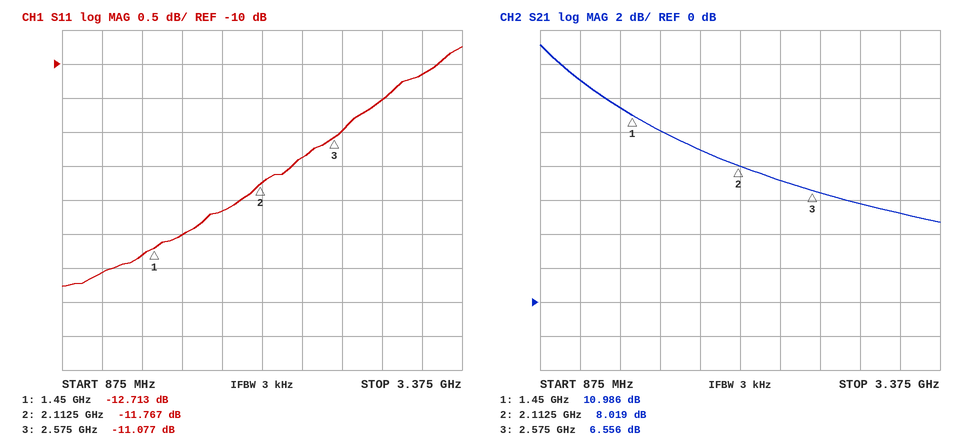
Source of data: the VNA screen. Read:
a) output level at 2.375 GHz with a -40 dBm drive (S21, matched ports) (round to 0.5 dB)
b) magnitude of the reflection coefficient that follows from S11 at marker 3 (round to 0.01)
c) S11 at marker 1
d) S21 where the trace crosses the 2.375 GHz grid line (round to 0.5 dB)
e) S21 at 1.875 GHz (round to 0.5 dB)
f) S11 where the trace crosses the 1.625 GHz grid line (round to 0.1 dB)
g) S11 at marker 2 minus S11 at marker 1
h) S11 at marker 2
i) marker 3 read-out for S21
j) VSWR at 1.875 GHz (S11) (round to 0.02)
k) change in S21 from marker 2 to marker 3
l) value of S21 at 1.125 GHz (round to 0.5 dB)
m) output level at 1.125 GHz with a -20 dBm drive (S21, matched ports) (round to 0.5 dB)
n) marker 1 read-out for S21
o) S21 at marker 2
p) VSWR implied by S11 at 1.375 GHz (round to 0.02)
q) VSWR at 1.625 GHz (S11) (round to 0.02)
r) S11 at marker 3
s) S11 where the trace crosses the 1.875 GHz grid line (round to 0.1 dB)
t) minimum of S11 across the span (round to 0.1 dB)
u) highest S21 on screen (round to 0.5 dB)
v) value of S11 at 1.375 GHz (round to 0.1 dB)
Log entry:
-33.0 dBm
0.28
-12.713 dB
7.0 dB
9.0 dB
-12.5 dB
0.946 dB
-11.767 dB
6.556 dB
1.66
-1.463 dB
13.0 dB
-7.0 dBm
10.986 dB
8.019 dB
1.60
1.62
-11.077 dB
-12.2 dB
-13.3 dB
15.0 dB
-12.8 dB
